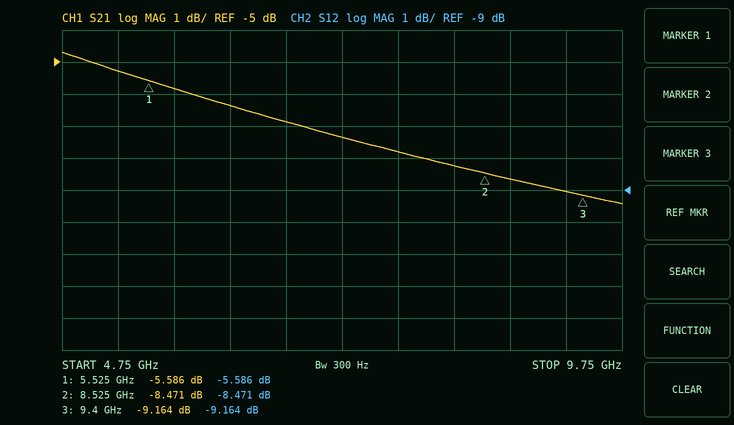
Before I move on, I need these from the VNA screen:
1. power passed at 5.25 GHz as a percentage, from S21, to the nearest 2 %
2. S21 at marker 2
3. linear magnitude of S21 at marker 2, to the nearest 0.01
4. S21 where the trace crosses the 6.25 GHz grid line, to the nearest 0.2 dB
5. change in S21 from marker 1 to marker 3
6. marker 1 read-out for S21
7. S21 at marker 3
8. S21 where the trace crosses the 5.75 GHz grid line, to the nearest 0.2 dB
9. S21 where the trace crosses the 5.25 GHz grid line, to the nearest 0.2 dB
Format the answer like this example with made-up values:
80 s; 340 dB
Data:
30 %; -8.471 dB; 0.38; -6.4 dB; -3.578 dB; -5.586 dB; -9.164 dB; -5.8 dB; -5.2 dB
